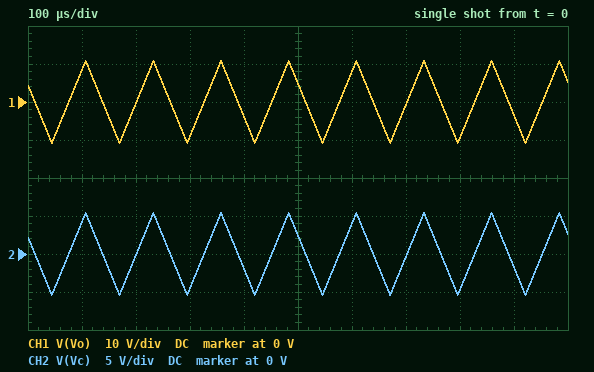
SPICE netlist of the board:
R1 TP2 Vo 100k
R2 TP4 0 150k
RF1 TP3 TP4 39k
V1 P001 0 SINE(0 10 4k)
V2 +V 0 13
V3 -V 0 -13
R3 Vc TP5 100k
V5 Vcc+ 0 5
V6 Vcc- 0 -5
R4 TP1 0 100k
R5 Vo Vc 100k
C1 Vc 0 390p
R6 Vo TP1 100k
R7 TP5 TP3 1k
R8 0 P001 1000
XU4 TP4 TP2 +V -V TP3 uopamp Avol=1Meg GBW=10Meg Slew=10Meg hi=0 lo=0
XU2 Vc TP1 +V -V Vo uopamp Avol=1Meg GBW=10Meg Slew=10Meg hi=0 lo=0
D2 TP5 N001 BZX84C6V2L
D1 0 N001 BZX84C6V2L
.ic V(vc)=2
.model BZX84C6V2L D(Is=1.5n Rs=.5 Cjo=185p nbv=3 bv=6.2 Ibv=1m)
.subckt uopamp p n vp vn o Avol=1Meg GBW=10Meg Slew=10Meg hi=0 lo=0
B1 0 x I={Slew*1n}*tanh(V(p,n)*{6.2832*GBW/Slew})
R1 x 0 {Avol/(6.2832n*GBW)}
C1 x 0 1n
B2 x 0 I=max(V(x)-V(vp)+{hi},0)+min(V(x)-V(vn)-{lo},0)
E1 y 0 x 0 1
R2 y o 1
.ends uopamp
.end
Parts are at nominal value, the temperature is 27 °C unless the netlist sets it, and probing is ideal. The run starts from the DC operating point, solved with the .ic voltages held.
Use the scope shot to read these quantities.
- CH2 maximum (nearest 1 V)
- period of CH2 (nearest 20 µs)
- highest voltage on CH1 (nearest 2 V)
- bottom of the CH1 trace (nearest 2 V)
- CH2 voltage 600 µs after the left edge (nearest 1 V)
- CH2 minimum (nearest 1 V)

5 V
120 µs
10 V
-10 V
4 V
-5 V
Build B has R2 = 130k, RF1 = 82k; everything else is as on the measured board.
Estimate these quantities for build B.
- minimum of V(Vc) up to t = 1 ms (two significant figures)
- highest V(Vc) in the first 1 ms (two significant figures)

-4.2 V
4.2 V
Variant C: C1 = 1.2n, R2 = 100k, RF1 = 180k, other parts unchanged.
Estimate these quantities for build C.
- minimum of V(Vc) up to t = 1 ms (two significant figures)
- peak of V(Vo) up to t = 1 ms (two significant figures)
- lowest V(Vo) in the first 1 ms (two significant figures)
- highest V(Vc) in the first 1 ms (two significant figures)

-2.4 V
4.8 V
-4.8 V
2.4 V
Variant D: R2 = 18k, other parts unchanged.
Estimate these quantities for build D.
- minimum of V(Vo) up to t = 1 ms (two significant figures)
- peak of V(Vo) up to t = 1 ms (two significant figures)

-4.5 V
4.5 V
